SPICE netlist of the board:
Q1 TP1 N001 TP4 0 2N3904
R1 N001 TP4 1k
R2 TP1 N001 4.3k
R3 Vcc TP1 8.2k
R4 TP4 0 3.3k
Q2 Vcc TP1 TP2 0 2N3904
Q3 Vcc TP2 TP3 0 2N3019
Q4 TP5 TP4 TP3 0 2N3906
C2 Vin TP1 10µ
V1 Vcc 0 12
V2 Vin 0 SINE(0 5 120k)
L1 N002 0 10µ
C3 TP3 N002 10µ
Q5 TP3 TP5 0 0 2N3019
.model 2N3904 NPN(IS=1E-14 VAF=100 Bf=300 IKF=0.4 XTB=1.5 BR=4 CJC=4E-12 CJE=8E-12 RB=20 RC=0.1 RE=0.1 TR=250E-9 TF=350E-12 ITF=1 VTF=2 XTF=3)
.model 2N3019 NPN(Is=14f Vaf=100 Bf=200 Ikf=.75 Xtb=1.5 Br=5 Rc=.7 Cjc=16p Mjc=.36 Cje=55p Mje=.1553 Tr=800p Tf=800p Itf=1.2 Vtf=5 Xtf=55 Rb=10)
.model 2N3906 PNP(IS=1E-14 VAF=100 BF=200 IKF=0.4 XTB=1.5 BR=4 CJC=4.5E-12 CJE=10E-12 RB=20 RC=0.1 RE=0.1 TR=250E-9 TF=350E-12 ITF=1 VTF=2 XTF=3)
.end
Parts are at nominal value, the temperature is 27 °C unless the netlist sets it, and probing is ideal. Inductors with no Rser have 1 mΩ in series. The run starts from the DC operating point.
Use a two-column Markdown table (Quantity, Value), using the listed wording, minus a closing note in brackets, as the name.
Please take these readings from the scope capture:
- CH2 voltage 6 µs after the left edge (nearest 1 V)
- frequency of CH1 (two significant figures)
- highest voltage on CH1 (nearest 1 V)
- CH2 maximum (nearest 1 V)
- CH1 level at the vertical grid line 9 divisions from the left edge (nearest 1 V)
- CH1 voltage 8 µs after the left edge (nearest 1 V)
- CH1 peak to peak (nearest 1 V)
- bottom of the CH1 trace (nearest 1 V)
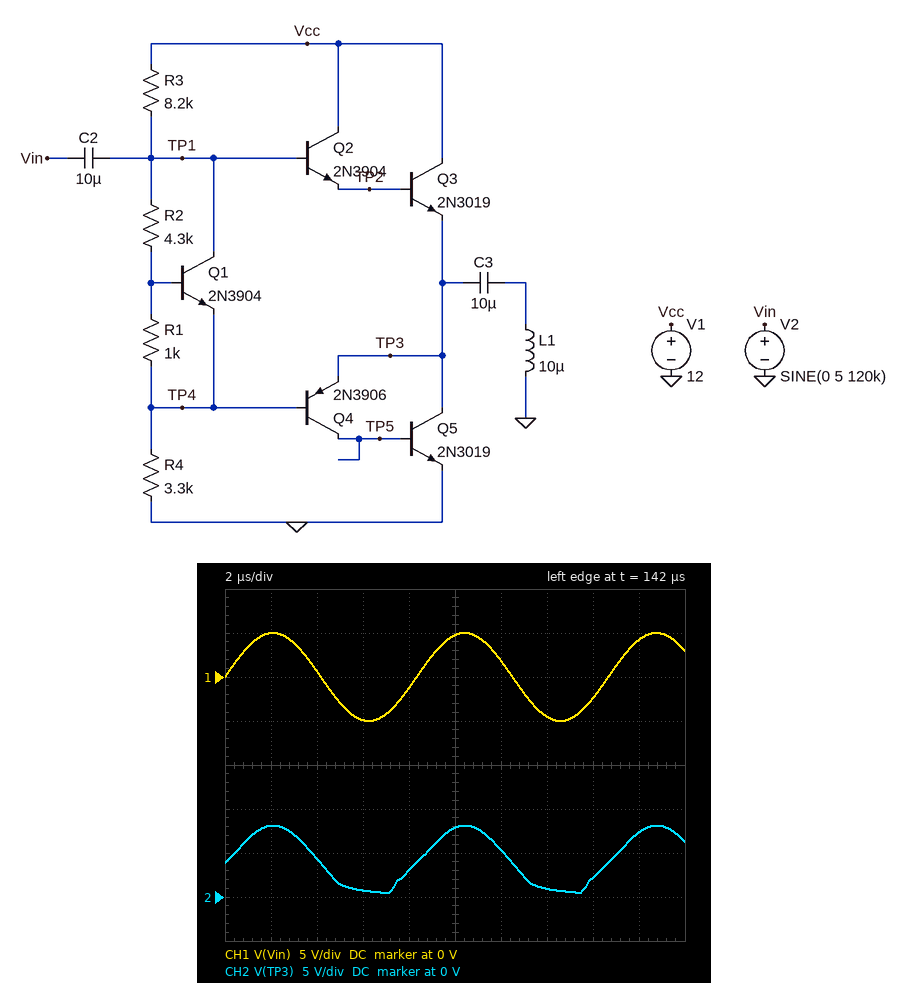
| Quantity | Value |
|---|---|
| CH2 voltage 6 µs after the left edge | 1 V |
| frequency of CH1 | 120 kHz |
| highest voltage on CH1 | 5 V |
| CH2 maximum | 8 V |
| CH1 level at the vertical grid line 9 divisions from the left edge | 4 V |
| CH1 voltage 8 µs after the left edge | -1 V |
| CH1 peak to peak | 10 V |
| bottom of the CH1 trace | -5 V |
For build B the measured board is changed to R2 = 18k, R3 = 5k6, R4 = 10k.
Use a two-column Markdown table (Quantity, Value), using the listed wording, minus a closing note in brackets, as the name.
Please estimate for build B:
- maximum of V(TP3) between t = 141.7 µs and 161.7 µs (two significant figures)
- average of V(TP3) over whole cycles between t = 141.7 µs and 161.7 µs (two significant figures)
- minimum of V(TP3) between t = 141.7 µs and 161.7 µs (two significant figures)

| Quantity | Value |
|---|---|
| maximum of V(TP3) between t = 141.7 µs and 161.7 µs | 9.4 V |
| average of V(TP3) over whole cycles between t = 141.7 µs and 161.7 µs | 6.5 V |
| minimum of V(TP3) between t = 141.7 µs and 161.7 µs | 2.5 V |
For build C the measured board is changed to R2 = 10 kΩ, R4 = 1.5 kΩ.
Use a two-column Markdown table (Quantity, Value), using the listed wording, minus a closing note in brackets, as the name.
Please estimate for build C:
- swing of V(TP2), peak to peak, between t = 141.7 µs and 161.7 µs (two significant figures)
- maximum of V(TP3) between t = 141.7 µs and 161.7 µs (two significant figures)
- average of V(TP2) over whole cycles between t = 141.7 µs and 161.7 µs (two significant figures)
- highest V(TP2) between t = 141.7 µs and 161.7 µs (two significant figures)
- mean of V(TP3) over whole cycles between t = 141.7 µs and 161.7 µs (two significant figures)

| Quantity | Value |
|---|---|
| swing of V(TP2), peak to peak, between t = 141.7 µs and 161.7 µs | 8.6 V |
| maximum of V(TP3) between t = 141.7 µs and 161.7 µs | 5.7 V |
| average of V(TP2) over whole cycles between t = 141.7 µs and 161.7 µs | 5.2 V |
| highest V(TP2) between t = 141.7 µs and 161.7 µs | 9.8 V |
| mean of V(TP3) over whole cycles between t = 141.7 µs and 161.7 µs | 3.1 V |
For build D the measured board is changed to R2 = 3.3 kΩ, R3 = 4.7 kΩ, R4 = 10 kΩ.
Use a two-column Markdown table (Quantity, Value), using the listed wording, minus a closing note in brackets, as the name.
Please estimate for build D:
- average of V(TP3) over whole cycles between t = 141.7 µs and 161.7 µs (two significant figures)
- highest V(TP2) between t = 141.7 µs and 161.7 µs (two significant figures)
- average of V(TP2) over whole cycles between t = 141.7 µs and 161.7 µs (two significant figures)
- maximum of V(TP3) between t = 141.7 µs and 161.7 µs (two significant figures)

| Quantity | Value |
|---|---|
| average of V(TP3) over whole cycles between t = 141.7 µs and 161.7 µs | 7.4 V |
| highest V(TP2) between t = 141.7 µs and 161.7 µs | 12 V |
| average of V(TP2) over whole cycles between t = 141.7 µs and 161.7 µs | 8.4 V |
| maximum of V(TP3) between t = 141.7 µs and 161.7 µs | 11 V |
